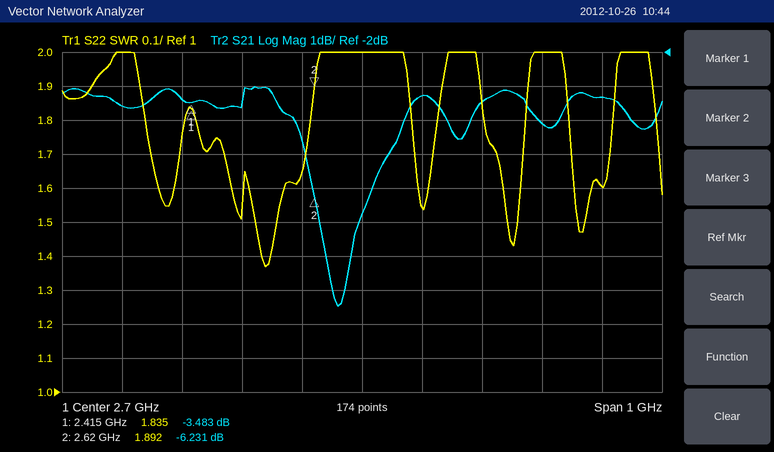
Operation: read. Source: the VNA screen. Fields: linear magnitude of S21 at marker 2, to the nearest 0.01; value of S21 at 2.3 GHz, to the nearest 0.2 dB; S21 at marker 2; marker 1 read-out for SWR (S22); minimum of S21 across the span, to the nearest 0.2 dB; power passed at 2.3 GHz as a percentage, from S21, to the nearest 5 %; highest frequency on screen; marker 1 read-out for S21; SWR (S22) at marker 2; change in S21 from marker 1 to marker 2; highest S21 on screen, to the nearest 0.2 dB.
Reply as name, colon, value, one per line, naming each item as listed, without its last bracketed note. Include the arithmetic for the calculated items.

linear magnitude of S21 at marker 2, to the nearest 0.01: 10^(-6.231/20) ≈ 0.49
value of S21 at 2.3 GHz, to the nearest 0.2 dB: -3.6 dB
S21 at marker 2: -6.231 dB
marker 1 read-out for SWR: 1.835
minimum of S21 across the span, to the nearest 0.2 dB: -9.4 dB
power passed at 2.3 GHz as a percentage, from S21, to the nearest 5 %: 10^(-3.6/10) ≈ 43.7 %, so 45 % to the nearest 5 %
highest frequency on screen: 3.2 GHz
marker 1 read-out for S21: -3.483 dB
SWR (S22) at marker 2: 1.892
change in S21 from marker 1 to marker 2: -6.231 − (-3.483) = -2.748 dB
highest S21 on screen, to the nearest 0.2 dB: -3.0 dB
